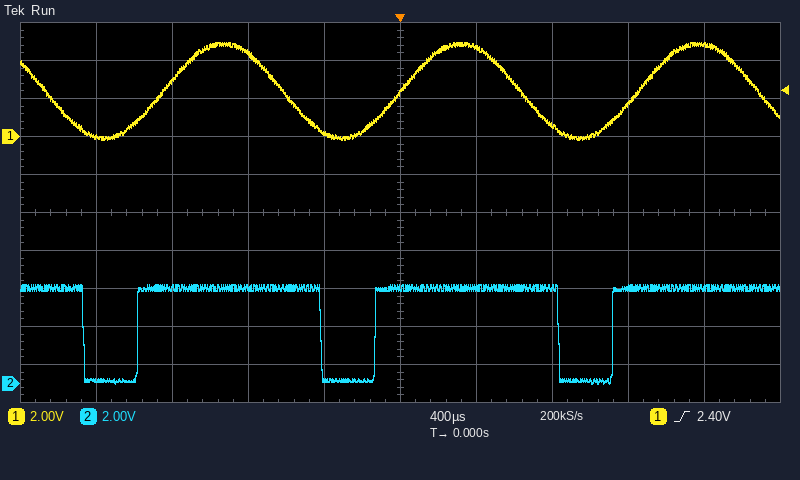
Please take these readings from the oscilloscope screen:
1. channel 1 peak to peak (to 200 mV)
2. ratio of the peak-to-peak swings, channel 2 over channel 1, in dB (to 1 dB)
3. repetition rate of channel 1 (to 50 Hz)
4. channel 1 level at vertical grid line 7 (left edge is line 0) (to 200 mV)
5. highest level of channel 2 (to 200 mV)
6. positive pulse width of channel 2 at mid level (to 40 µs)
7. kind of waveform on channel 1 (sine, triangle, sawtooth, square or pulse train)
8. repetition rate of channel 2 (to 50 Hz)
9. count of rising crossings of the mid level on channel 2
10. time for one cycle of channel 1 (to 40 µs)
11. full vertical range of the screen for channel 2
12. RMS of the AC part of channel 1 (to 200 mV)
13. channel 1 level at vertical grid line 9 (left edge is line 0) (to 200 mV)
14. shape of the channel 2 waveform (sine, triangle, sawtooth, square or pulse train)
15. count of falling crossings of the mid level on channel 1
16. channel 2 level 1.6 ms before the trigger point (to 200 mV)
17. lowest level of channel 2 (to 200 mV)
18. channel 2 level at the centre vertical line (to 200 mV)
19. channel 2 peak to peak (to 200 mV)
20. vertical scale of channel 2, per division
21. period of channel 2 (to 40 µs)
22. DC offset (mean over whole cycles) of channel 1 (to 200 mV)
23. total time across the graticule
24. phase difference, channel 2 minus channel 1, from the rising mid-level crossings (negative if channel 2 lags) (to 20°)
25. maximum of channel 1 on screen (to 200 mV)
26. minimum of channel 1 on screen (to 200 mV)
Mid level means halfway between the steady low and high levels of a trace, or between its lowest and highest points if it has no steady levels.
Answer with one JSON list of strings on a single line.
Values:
["5.2 V", "0 dB", "800 Hz", "600 mV", "5.2 V", "960 µs", "sine", "800 Hz", "3", "1.24 ms", "20 V", "1.8 V", "4.8 V", "pulse train", "4", "200 mV", "0.0 V", "5.0 V", "5.2 V", "2 V", "1.24 ms", "2.4 V", "4 ms", "+40°", "5.0 V", "-200 mV"]
